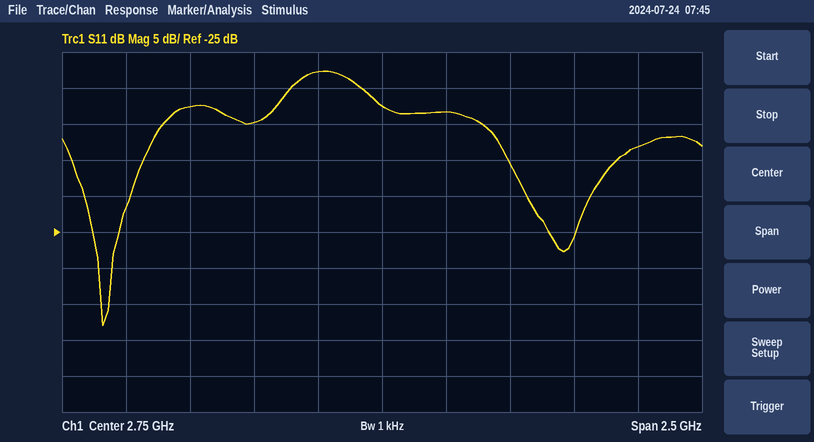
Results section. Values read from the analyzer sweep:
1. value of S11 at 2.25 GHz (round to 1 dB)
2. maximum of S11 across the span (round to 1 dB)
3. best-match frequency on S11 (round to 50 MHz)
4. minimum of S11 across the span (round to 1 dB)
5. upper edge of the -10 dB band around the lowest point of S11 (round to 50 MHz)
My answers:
-10 dB
-3 dB
1.65 GHz
-38 dB
1.90 GHz
